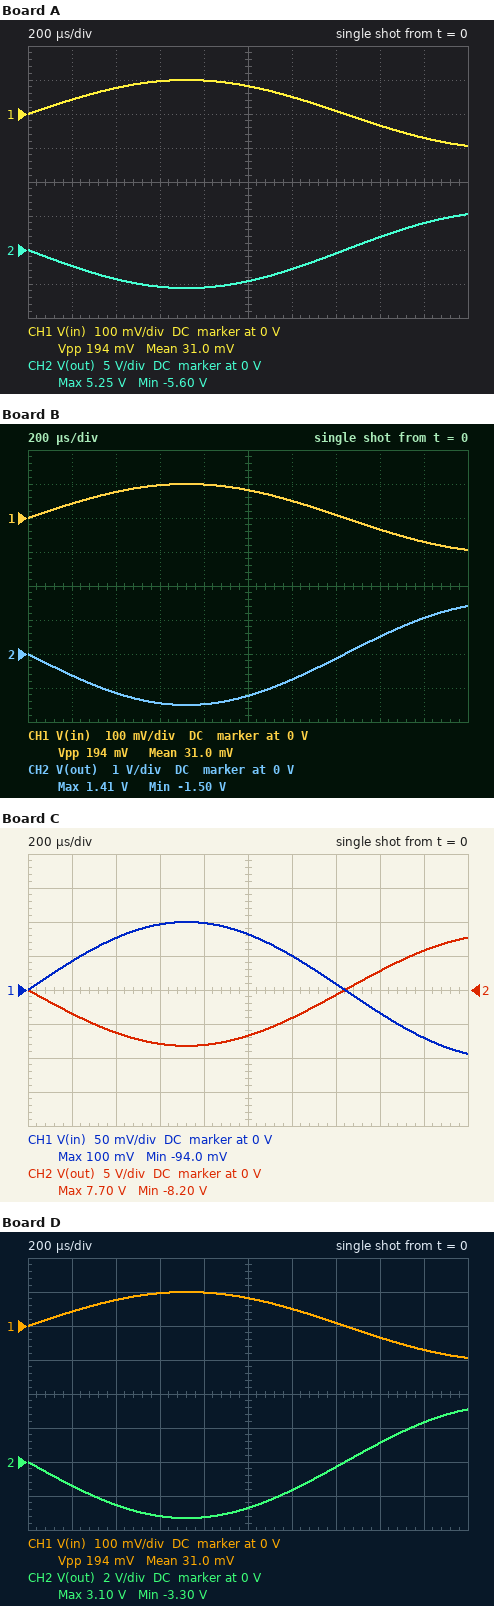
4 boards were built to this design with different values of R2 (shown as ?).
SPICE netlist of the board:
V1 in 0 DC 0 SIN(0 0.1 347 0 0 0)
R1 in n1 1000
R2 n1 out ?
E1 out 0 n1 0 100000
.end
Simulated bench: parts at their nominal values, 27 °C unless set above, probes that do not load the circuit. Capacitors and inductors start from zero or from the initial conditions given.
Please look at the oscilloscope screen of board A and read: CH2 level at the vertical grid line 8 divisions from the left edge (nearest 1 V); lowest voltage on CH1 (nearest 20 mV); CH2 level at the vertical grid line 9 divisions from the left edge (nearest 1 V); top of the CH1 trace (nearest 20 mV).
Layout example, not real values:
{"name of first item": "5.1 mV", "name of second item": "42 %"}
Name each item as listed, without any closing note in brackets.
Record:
{"CH2 level at the vertical grid line 8 divisions from the left edge": "2 V", "lowest voltage on CH1": "-100 mV", "CH2 level at the vertical grid line 9 divisions from the left edge": "4 V", "top of the CH1 trace": "100 mV"}
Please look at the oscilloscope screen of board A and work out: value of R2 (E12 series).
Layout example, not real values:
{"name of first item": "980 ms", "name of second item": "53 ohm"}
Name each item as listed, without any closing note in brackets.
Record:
{"value of R2": "56 kΩ"}
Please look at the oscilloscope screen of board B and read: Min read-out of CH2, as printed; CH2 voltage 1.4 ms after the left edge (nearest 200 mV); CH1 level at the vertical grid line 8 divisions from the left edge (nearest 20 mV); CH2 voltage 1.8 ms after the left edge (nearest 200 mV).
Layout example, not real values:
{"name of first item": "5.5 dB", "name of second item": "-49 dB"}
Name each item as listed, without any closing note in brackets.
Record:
{"Min read-out of CH2, as printed": "-1.50 V", "CH2 voltage 1.4 ms after the left edge": "-200 mV", "CH1 level at the vertical grid line 8 divisions from the left edge": "-40 mV", "CH2 voltage 1.8 ms after the left edge": "1.0 V"}
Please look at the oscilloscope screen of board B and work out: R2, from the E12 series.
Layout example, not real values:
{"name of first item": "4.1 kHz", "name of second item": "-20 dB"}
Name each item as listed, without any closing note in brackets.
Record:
{"R2, from the E12 series": "15 kΩ"}
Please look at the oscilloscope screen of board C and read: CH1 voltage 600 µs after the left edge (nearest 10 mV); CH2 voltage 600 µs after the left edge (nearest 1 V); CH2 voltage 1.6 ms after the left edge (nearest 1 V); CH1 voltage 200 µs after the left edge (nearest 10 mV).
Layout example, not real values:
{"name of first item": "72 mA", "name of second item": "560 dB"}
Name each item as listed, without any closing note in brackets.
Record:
{"CH1 voltage 600 µs after the left edge": "100 mV", "CH2 voltage 600 µs after the left edge": "-8 V", "CH2 voltage 1.6 ms after the left edge": "3 V", "CH1 voltage 200 µs after the left edge": "40 mV"}
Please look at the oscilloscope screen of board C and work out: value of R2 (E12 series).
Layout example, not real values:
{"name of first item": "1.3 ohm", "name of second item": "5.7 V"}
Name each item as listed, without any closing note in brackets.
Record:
{"value of R2": "82 kΩ"}
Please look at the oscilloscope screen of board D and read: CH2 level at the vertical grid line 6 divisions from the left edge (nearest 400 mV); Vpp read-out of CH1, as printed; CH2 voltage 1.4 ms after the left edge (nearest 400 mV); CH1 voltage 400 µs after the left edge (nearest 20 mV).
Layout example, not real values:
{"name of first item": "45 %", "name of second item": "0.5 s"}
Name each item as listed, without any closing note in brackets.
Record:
{"CH2 level at the vertical grid line 6 divisions from the left edge": "-1.6 V", "Vpp read-out of CH1, as printed": "194 mV", "CH2 voltage 1.4 ms after the left edge": "-400 mV", "CH1 voltage 400 µs after the left edge": "80 mV"}
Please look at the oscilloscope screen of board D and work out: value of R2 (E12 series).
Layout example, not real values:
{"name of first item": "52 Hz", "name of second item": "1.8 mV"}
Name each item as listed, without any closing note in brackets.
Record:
{"value of R2": "33 kΩ"}
